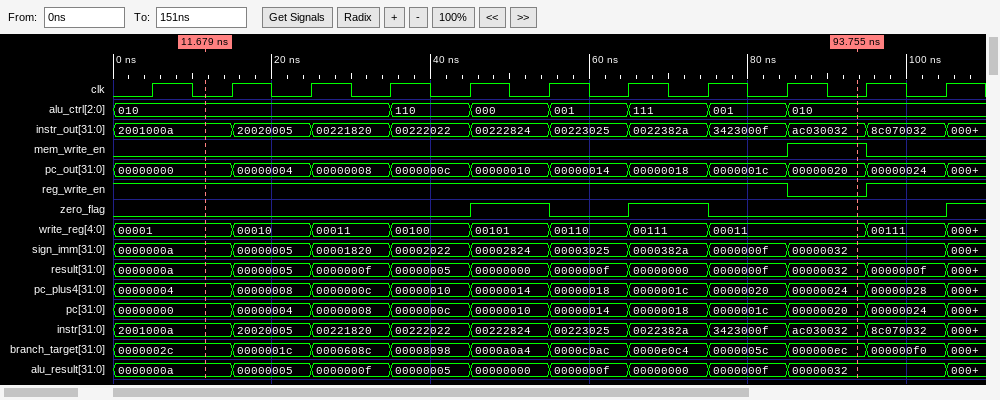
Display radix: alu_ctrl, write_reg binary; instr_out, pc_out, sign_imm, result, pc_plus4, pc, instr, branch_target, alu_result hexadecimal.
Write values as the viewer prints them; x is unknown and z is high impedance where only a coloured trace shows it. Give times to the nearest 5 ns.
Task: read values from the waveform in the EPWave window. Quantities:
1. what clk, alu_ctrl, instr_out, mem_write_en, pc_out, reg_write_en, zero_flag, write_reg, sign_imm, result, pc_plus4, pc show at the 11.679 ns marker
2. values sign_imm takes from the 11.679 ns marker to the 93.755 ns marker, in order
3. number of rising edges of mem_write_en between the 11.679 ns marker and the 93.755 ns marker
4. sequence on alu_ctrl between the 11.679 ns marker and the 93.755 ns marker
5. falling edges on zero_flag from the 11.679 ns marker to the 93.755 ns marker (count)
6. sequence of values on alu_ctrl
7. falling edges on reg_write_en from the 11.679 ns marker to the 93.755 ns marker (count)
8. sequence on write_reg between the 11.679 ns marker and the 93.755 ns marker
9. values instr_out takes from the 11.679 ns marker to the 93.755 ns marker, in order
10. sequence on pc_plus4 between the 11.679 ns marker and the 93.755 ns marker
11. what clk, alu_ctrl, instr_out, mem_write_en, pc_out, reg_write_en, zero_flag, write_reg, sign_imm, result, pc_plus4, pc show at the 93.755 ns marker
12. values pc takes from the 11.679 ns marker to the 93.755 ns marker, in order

clk=0, alu_ctrl=010, instr_out=2001000a, mem_write_en=0, pc_out=00000000, reg_write_en=1, zero_flag=0, write_reg=00001, sign_imm=0000000a, result=0000000a, pc_plus4=00000004, pc=00000000
0000000a, 00000005, 00001820, 00002022, 00002824, 00003025, 0000382a, 0000000f, 00000032
1
010, 110, 000, 001, 111, 001, 010
2
010, 110, 000, 001, 111, 001, 010
1
00001, 00010, 00011, 00100, 00101, 00110, 00111, 00011
2001000a, 20020005, 00221820, 00222022, 00222824, 00223025, 0022382a, 3423000f, ac030032
00000004, 00000008, 0000000c, 00000010, 00000014, 00000018, 0000001c, 00000020, 00000024
clk=0, alu_ctrl=010, instr_out=ac030032, mem_write_en=1, pc_out=00000020, reg_write_en=0, zero_flag=0, write_reg=00011, sign_imm=00000032, result=00000032, pc_plus4=00000024, pc=00000020
00000000, 00000004, 00000008, 0000000c, 00000010, 00000014, 00000018, 0000001c, 00000020
